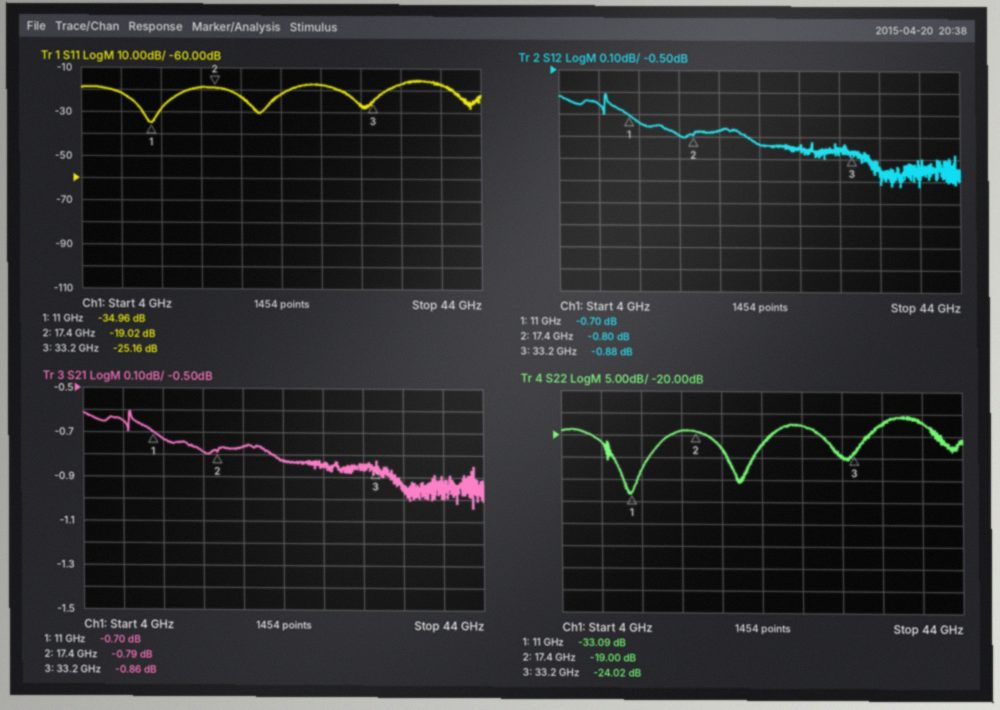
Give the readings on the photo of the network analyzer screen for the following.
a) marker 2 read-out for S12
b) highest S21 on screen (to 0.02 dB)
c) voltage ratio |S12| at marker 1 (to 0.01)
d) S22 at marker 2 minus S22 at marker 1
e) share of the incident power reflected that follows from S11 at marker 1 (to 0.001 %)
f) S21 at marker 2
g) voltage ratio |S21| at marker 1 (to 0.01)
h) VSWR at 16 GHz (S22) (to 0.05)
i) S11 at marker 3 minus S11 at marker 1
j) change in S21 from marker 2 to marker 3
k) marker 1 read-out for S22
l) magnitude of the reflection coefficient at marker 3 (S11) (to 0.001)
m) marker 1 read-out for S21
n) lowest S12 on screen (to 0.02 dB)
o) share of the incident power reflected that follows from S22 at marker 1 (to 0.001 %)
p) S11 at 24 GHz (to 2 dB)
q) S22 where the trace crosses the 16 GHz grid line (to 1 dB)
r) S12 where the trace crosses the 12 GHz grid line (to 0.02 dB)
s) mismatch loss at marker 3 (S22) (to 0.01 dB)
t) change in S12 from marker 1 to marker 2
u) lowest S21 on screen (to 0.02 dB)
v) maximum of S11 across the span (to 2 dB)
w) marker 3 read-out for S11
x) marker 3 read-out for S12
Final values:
-0.80 dB
-0.60 dB
0.92
14.09 dB
0.032 %
-0.79 dB
0.92
1.25
9.80 dB
-0.07 dB
-33.09 dB
0.055
-0.70 dB
-1.02 dB
0.049 %
-22 dB
-19 dB
-0.74 dB
0.02 dB
-0.10 dB
-1.04 dB
-16 dB
-25.16 dB
-0.88 dB
